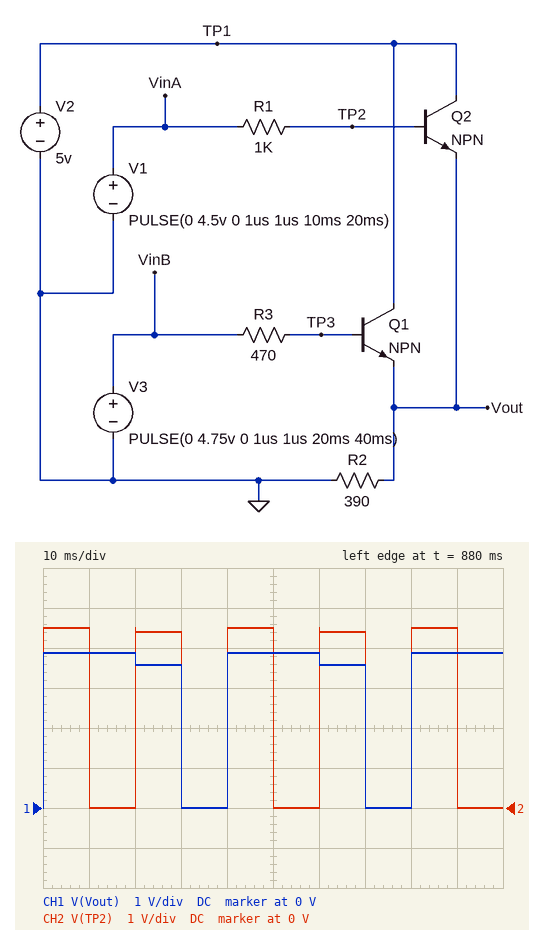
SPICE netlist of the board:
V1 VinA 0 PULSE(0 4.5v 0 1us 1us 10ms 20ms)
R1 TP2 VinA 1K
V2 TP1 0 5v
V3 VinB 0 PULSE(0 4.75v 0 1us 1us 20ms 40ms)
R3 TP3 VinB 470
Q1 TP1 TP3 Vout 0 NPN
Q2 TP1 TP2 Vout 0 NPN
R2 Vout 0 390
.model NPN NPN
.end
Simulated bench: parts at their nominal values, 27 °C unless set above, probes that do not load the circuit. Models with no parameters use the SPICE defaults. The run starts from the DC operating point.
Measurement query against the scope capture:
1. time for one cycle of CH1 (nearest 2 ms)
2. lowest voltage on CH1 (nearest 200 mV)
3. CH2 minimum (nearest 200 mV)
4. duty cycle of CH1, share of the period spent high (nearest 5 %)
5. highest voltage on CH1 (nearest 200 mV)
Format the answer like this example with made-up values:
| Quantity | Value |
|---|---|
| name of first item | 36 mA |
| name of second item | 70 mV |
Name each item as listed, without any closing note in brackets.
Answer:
| Quantity | Value |
|---|---|
| time for one cycle of CH1 | 40 ms |
| lowest voltage on CH1 | 0 V |
| CH2 minimum | 0 V |
| duty cycle of CH1, share of the period spent high | 75 % |
| highest voltage on CH1 | 3.8 V |
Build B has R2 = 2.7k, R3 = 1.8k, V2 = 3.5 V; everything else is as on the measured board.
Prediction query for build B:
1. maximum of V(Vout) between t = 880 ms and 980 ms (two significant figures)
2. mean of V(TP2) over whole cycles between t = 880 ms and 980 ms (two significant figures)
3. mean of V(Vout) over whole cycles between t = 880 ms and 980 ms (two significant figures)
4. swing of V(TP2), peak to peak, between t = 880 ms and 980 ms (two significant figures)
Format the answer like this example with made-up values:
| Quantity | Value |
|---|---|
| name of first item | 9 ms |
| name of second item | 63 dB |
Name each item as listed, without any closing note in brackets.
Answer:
| Quantity | Value |
|---|---|
| maximum of V(Vout) between t = 880 ms and 980 ms | 3.5 V |
| mean of V(TP2) over whole cycles between t = 880 ms and 980 ms | 2.1 V |
| mean of V(Vout) over whole cycles between t = 880 ms and 980 ms | 2.6 V |
| swing of V(TP2), peak to peak, between t = 880 ms and 980 ms | 4.2 V |
